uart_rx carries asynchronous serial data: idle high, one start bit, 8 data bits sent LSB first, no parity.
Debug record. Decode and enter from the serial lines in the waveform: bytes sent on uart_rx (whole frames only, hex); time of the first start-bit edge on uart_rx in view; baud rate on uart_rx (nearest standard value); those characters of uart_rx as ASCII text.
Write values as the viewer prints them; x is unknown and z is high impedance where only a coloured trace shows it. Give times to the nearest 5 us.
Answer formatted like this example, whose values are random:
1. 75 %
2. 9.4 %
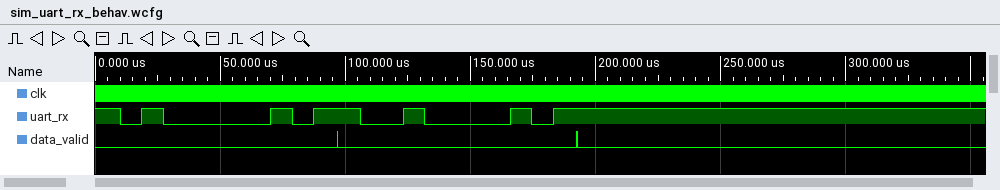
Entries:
1. 41, 42
2. 10 us
3. 115200 baud
4. "AB"
